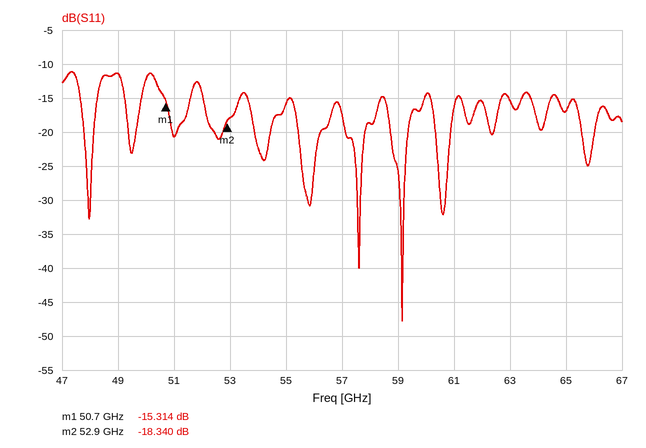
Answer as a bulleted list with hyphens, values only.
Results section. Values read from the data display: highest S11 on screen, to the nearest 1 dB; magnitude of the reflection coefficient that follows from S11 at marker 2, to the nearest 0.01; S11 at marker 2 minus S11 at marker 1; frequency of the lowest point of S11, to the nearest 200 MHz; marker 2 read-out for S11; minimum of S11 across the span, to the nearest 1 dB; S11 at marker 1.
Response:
- -11 dB
- 0.12
- -3.026 dB
- 59.2 GHz
- -18.340 dB
- -48 dB
- -15.314 dB
